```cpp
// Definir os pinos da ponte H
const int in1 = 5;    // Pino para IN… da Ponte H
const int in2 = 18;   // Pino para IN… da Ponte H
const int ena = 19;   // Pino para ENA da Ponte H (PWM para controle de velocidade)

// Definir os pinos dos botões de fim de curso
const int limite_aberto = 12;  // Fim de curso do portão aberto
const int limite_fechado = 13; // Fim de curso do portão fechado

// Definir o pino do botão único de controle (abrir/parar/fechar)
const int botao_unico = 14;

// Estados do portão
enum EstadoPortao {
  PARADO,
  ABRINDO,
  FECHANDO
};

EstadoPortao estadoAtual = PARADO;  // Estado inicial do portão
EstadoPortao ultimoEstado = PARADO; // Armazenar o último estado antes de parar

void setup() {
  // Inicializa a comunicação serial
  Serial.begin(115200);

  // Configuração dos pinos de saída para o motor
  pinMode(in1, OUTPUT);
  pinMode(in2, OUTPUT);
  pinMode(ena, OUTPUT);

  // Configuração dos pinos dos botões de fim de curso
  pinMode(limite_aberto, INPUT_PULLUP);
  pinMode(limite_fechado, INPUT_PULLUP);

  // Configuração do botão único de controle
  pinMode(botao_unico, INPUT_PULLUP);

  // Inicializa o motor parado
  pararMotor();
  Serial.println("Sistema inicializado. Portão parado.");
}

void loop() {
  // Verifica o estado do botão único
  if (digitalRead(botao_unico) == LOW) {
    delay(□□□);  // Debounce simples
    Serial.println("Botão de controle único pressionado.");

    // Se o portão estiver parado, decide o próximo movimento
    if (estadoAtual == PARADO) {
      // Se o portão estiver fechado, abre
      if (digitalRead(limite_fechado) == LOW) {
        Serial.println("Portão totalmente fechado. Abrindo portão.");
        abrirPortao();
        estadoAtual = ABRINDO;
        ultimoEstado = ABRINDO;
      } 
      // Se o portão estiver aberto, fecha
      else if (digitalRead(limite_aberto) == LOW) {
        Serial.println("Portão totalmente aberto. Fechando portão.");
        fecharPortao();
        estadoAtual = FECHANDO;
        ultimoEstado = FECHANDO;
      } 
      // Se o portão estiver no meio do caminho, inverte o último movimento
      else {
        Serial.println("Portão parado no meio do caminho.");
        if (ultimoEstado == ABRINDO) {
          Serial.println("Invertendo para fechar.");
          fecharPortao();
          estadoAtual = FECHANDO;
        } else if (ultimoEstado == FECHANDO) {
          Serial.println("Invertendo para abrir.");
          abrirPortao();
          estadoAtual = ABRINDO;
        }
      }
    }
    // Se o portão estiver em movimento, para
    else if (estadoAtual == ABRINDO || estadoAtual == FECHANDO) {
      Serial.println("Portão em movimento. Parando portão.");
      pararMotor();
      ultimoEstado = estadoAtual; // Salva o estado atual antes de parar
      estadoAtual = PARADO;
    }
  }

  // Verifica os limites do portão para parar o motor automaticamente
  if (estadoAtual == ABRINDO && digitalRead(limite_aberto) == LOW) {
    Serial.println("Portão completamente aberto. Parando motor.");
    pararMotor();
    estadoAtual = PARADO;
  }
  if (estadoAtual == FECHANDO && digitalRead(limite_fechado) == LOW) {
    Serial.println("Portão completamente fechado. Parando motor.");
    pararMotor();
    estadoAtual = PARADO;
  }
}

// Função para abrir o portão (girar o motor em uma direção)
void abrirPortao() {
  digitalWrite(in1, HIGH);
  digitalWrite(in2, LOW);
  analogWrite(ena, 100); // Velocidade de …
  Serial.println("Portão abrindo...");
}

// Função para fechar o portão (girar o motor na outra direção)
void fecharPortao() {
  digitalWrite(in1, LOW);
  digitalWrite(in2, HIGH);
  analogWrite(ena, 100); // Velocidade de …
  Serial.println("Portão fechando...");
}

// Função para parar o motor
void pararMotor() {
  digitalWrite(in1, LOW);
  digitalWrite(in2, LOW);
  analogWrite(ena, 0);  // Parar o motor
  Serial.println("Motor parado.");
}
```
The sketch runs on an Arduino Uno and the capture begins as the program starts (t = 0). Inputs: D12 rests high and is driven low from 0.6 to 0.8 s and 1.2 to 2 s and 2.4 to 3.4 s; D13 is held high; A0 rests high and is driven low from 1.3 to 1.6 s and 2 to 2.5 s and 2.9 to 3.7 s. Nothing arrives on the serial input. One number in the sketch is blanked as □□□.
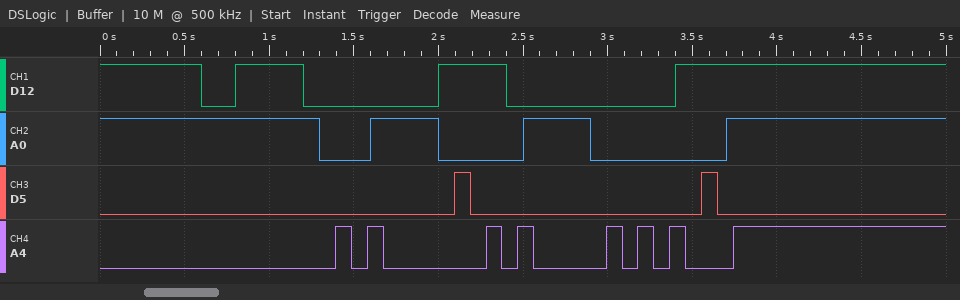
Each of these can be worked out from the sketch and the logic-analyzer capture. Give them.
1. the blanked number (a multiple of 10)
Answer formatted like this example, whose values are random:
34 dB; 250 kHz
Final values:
90
